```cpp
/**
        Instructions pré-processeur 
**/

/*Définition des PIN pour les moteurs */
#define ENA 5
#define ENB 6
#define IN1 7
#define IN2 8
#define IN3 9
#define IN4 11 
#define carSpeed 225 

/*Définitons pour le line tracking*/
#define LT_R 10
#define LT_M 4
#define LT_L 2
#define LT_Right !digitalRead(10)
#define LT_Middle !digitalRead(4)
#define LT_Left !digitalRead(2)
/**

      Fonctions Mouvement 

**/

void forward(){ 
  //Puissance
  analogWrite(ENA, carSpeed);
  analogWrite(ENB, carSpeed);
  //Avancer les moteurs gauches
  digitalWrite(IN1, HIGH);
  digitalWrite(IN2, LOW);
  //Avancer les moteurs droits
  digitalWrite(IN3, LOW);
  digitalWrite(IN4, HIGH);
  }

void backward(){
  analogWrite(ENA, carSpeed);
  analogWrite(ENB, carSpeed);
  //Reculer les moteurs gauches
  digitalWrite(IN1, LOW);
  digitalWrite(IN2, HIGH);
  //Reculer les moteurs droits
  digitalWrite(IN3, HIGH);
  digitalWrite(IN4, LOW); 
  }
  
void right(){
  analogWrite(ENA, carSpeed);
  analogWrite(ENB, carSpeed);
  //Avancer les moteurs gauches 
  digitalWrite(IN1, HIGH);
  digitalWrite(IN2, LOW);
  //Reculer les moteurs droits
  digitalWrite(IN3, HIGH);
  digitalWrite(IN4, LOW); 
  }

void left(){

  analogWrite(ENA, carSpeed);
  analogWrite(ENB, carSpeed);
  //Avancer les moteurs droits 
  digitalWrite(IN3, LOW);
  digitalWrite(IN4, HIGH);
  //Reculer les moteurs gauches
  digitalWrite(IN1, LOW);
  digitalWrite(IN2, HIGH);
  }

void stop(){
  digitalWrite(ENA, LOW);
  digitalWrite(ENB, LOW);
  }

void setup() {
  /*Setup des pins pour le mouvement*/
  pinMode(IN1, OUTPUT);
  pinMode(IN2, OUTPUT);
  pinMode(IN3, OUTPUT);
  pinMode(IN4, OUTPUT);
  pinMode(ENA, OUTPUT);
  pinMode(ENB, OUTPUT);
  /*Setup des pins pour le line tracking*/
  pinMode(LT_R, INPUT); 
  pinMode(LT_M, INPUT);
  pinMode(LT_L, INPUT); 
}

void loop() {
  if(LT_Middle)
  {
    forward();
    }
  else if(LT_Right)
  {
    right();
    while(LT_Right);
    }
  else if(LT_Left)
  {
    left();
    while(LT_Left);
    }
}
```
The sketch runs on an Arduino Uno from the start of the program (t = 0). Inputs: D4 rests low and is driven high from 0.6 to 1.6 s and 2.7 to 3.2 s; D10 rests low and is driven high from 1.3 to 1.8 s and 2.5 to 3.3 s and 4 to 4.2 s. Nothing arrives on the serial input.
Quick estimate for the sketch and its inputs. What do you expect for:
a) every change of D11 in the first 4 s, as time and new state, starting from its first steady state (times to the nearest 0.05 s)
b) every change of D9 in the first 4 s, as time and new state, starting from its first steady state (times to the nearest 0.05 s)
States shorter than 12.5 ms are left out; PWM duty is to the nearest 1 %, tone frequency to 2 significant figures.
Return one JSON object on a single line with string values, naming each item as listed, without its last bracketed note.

{"every change of D11 in the first 4 s, as time and new state, starting from its first steady state": "0 s high; 0.6 s low; 1.3 s high", "every change of D9 in the first 4 s, as time and new state, starting from its first steady state": "0 s low; 0.6 s high; 1.3 s low"}
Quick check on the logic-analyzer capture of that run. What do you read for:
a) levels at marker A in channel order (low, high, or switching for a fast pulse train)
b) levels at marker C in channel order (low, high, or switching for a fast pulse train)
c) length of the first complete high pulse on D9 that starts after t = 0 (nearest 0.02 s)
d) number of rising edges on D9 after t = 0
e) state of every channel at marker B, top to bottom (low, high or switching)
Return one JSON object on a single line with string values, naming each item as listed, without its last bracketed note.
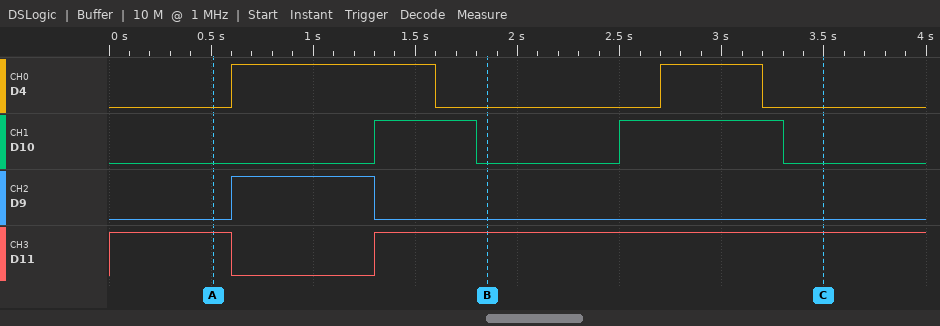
{"levels at marker A in channel order": "D4 low, D10 low, D9 low, D11 high", "levels at marker C in channel order": "D4 low, D10 low, D9 low, D11 high", "length of the first complete high pulse on D9 that starts after t = 0": "0.70 s", "number of rising edges on D9 after t = 0": "1", "state of every channel at marker B, top to bottom": "D4 low, D10 low, D9 low, D11 high"}
